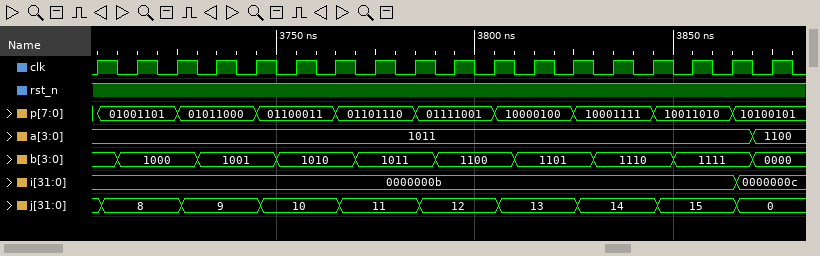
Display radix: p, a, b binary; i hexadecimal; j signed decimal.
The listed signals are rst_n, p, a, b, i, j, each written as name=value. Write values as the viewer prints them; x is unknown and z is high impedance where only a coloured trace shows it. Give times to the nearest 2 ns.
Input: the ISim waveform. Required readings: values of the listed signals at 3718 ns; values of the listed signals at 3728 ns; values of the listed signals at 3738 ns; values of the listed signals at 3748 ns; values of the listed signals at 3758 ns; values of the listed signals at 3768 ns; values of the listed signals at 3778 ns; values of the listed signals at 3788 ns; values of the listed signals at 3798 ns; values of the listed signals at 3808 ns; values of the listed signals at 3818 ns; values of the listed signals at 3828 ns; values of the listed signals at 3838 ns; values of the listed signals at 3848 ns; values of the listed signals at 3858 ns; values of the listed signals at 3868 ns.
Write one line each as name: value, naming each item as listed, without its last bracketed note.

values of the listed signals at 3718 ns: rst_n=1, p=01001101, a=1011, b=1000, i=0000000b, j=8
values of the listed signals at 3728 ns: rst_n=1, p=01011000, a=1011, b=1000, i=0000000b, j=9
values of the listed signals at 3738 ns: rst_n=1, p=01011000, a=1011, b=1001, i=0000000b, j=9
values of the listed signals at 3748 ns: rst_n=1, p=01100011, a=1011, b=1001, i=0000000b, j=10
values of the listed signals at 3758 ns: rst_n=1, p=01100011, a=1011, b=1010, i=0000000b, j=10
values of the listed signals at 3768 ns: rst_n=1, p=01101110, a=1011, b=1010, i=0000000b, j=11
values of the listed signals at 3778 ns: rst_n=1, p=01101110, a=1011, b=1011, i=0000000b, j=11
values of the listed signals at 3788 ns: rst_n=1, p=01111001, a=1011, b=1011, i=0000000b, j=12
values of the listed signals at 3798 ns: rst_n=1, p=01111001, a=1011, b=1100, i=0000000b, j=12
values of the listed signals at 3808 ns: rst_n=1, p=10000100, a=1011, b=1100, i=0000000b, j=13
values of the listed signals at 3818 ns: rst_n=1, p=10000100, a=1011, b=1101, i=0000000b, j=13
values of the listed signals at 3828 ns: rst_n=1, p=10001111, a=1011, b=1101, i=0000000b, j=14
values of the listed signals at 3838 ns: rst_n=1, p=10001111, a=1011, b=1110, i=0000000b, j=14
values of the listed signals at 3848 ns: rst_n=1, p=10011010, a=1011, b=1110, i=0000000b, j=15
values of the listed signals at 3858 ns: rst_n=1, p=10011010, a=1011, b=1111, i=0000000b, j=15
values of the listed signals at 3868 ns: rst_n=1, p=10100101, a=1011, b=1111, i=0000000c, j=0
